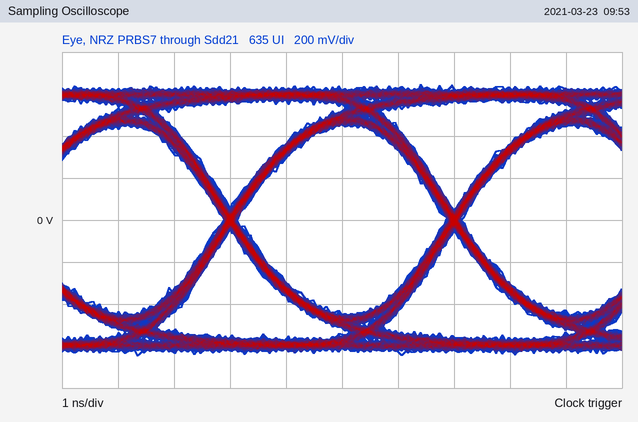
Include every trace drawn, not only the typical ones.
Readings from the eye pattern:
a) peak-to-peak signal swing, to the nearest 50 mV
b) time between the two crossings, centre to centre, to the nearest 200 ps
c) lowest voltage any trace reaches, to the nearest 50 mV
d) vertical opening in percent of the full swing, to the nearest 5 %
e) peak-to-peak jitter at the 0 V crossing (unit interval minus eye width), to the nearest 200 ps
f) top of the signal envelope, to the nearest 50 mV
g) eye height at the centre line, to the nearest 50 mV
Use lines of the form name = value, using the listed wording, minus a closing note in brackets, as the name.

peak-to-peak signal swing, to the nearest 50 mV = 1.30 V
time between the two crossings, centre to centre, to the nearest 200 ps = 4.0 ns
lowest voltage any trace reaches, to the nearest 50 mV = -650 mV
vertical opening in percent of the full swing, to the nearest 5 % = 70 %
peak-to-peak jitter at the 0 V crossing (unit interval minus eye width), to the nearest 200 ps = 200 ps
top of the signal envelope, to the nearest 50 mV = 650 mV
eye height at the centre line, to the nearest 50 mV = 900 mV
